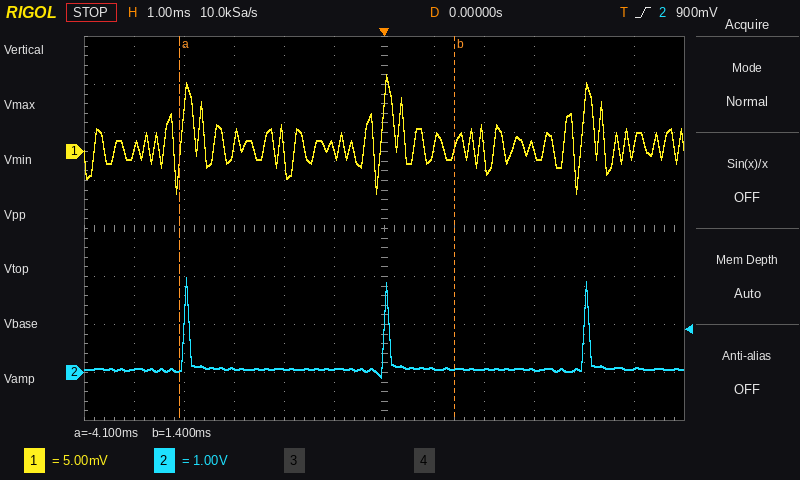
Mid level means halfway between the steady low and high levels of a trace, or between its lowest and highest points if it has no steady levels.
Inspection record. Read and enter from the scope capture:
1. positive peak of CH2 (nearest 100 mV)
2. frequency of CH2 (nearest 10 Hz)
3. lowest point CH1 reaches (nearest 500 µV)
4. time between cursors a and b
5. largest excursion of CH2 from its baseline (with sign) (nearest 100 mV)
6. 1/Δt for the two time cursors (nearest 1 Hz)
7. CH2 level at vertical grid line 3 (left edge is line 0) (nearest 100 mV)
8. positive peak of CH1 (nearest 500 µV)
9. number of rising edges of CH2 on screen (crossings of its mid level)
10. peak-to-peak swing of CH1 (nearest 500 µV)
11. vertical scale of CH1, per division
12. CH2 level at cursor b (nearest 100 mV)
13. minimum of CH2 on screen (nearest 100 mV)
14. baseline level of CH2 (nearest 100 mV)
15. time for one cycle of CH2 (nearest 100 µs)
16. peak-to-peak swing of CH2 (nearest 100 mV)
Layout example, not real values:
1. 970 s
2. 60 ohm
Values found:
1. 2.0 V
2. 250 Hz
3. -4.5 mV
4. 5.5 ms
5. +1.9 V
6. 182 Hz
7. 100 mV
8. 8.0 mV
9. 3
10. 12.5 mV
11. 5 mV
12. 100 mV
13. -100 mV
14. 100 mV
15. 4.0 ms
16. 2.1 V
